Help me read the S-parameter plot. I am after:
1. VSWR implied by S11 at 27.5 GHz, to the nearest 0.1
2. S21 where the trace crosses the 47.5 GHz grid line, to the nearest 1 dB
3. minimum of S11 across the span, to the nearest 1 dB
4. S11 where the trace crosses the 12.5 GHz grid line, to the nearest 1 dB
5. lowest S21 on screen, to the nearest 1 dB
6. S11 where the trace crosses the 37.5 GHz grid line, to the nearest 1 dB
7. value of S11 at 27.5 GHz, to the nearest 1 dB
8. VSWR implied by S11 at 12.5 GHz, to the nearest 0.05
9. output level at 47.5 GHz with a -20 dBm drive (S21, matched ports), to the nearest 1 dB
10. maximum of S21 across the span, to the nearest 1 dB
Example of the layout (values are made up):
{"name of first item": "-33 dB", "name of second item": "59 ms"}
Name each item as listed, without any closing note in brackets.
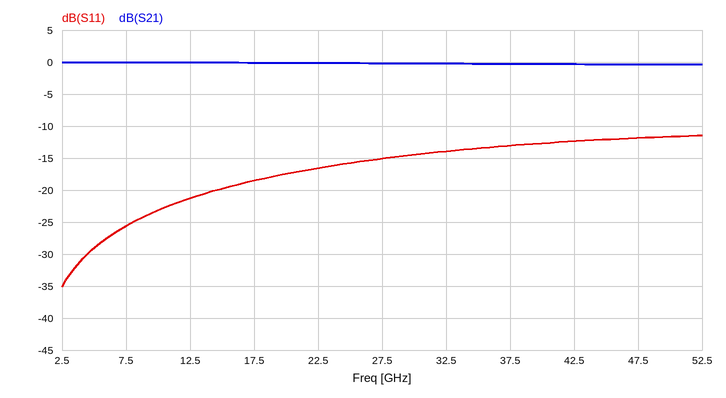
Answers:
{"VSWR implied by S11 at 27.5 GHz, to the nearest 0.1": "1.4", "S21 where the trace crosses the 47.5 GHz grid line, to the nearest 1 dB": "0 dB", "minimum of S11 across the span, to the nearest 1 dB": "-35 dB", "S11 where the trace crosses the 12.5 GHz grid line, to the nearest 1 dB": "-21 dB", "lowest S21 on screen, to the nearest 1 dB": "0 dB", "S11 where the trace crosses the 37.5 GHz grid line, to the nearest 1 dB": "-13 dB", "value of S11 at 27.5 GHz, to the nearest 1 dB": "-15 dB", "VSWR implied by S11 at 12.5 GHz, to the nearest 0.05": "1.20", "output level at 47.5 GHz with a -20 dBm drive (S21, matched ports), to the nearest 1 dB": "-20 dBm", "maximum of S21 across the span, to the nearest 1 dB": "0 dB"}
